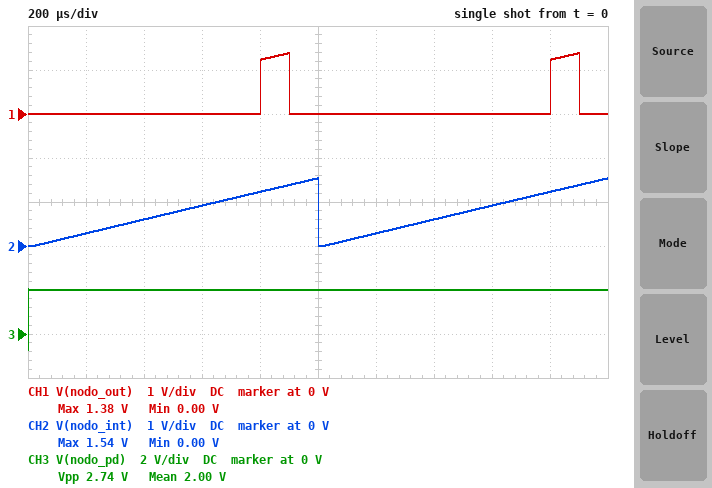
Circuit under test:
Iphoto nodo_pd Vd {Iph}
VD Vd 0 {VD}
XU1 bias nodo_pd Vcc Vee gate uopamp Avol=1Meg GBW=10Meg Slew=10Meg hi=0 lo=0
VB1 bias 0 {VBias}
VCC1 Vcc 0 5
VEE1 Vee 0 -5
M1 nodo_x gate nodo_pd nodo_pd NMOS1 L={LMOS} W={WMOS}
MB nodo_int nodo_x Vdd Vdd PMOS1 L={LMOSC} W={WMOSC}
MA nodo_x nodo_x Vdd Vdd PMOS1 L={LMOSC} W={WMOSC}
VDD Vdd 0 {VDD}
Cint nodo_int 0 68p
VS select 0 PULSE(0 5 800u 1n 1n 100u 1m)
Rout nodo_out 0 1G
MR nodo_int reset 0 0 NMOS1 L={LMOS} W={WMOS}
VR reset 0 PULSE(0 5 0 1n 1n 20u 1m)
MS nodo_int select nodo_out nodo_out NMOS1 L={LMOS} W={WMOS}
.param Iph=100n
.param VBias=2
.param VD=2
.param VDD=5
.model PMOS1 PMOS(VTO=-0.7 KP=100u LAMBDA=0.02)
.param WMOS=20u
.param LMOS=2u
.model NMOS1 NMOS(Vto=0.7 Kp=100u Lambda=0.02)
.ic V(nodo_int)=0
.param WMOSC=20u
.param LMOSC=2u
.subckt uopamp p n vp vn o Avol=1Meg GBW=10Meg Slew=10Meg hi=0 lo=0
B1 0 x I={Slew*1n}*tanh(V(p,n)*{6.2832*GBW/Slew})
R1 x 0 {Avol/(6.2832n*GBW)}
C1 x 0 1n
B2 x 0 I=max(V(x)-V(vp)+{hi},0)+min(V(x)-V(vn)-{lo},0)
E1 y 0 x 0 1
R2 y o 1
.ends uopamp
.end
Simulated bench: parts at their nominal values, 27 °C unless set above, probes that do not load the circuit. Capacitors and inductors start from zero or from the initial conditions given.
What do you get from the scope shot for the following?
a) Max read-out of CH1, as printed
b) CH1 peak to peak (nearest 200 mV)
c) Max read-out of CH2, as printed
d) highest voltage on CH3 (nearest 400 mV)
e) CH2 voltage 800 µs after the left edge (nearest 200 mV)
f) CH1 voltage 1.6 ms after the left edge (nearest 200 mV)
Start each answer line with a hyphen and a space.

- 1.38 V
- 1.4 V
- 1.54 V
- 2.0 V
- 1.2 V
- 0 V
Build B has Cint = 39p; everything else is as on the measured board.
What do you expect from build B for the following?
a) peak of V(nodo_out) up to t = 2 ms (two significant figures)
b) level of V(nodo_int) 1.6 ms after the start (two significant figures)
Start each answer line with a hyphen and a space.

- 2.4 V
- 1.6 V
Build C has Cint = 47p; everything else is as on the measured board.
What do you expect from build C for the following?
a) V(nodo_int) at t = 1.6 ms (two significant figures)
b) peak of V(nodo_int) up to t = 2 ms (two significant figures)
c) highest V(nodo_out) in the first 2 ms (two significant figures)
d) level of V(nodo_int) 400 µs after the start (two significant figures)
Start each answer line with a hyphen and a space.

- 1.3 V
- 2.2 V
- 2.0 V
- 870 mV
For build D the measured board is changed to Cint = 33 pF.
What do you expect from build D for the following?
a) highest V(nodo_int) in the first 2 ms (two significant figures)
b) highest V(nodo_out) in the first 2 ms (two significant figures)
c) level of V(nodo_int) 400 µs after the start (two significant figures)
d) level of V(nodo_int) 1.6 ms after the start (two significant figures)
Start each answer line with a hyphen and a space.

- 3.1 V
- 2.8 V
- 1.2 V
- 1.9 V
